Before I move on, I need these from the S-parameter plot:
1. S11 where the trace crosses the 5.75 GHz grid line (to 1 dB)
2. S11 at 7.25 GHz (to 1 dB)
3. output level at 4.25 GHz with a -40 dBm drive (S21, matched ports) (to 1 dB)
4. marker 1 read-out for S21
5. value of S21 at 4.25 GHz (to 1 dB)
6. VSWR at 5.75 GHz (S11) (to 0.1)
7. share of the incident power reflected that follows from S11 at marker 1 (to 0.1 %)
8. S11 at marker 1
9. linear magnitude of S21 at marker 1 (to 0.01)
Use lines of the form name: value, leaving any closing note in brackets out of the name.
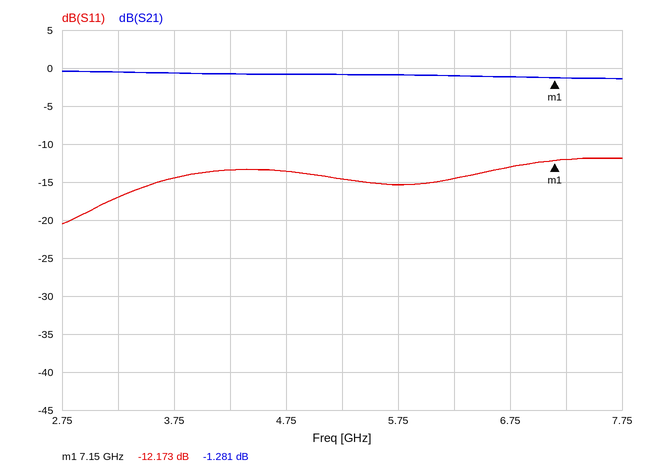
S11 where the trace crosses the 5.75 GHz grid line: -15 dB
S11 at 7.25 GHz: -12 dB
output level at 4.25 GHz with a -40 dBm drive (S21, matched ports): -41 dBm
marker 1 read-out for S21: -1.281 dB
value of S21 at 4.25 GHz: -1 dB
VSWR at 5.75 GHz (S11): 1.4
share of the incident power reflected that follows from S11 at marker 1: 6.1 %
S11 at marker 1: -12.173 dB
linear magnitude of S21 at marker 1: 0.86
